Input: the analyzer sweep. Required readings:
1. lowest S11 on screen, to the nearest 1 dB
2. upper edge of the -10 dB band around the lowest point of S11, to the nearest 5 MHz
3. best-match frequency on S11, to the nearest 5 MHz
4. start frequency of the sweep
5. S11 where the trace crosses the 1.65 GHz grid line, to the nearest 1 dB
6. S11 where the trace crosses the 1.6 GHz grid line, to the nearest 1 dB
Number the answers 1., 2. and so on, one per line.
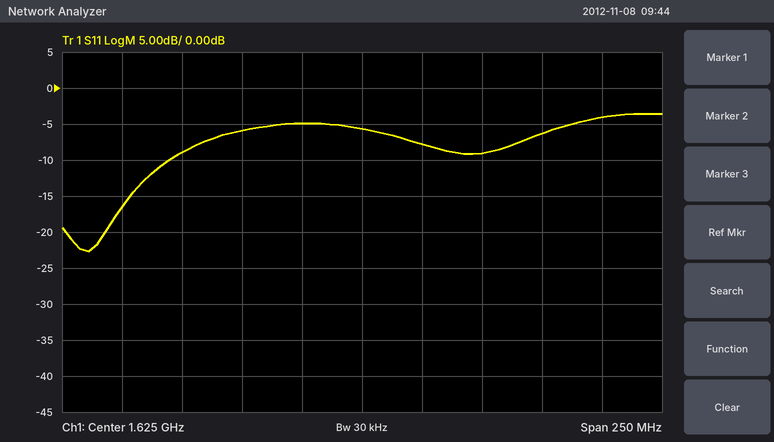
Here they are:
1. -23 dB
2. 1.545 GHz
3. 1.510 GHz
4. 1.5 GHz
5. -8 dB
6. -5 dB
